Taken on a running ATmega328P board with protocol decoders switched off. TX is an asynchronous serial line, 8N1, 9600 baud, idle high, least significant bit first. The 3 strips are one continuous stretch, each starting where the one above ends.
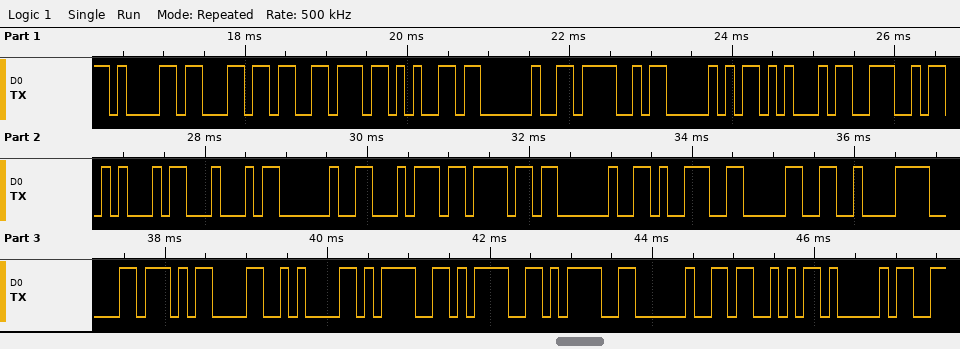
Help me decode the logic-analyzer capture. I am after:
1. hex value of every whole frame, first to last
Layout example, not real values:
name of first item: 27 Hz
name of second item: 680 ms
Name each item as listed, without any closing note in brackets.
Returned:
hex value of every whole frame, first to last: 0x61 0x6C 0x76 0x65 0x20 0x4F 0x50 0x45 0x4E 0x45 0x44 0x20 0x74 0x6F 0x20 0x39 0x30 0xC2 0xB0 0x0D 0x0A 0x3D 0x3D 0x3D 0x20 0x53 0x41
